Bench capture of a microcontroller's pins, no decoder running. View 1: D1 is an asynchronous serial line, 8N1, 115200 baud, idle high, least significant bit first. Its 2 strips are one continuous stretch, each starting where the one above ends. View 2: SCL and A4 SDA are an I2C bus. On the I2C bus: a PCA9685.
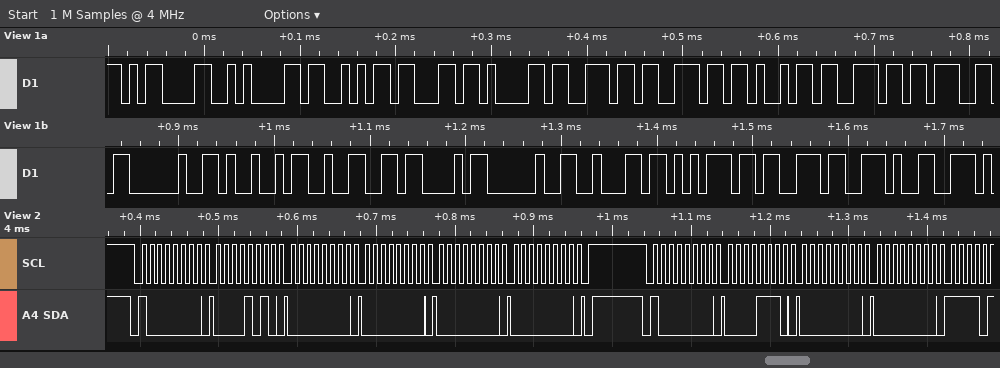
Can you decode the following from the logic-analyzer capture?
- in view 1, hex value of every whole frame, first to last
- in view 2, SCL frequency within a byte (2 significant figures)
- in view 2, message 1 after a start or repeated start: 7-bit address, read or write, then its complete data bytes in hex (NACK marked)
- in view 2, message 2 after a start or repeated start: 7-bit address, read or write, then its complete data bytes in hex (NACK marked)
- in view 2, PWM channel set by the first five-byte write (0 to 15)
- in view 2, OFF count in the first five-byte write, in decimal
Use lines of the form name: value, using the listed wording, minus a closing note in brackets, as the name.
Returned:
in view 1, hex value of every whole frame, first to last: 0D 0A 53 63 61 6E 6E 69 6E 67 20 49 32 43 20 62 75 73 2E
in view 2, SCL frequency within a byte: 100 kHz
in view 2, message 1 after a start or repeated start: 7-bit address, read or write, then its complete data bytes in hex: 0x40 write: 0A 00 00 00 00
in view 2, message 2 after a start or repeated start: 7-bit address, read or write, then its complete data bytes in hex: 0x40 write: 0E 00 00
in view 2, PWM channel set by the first five-byte write: 1
in view 2, OFF count in the first five-byte write, in decimal: 0
